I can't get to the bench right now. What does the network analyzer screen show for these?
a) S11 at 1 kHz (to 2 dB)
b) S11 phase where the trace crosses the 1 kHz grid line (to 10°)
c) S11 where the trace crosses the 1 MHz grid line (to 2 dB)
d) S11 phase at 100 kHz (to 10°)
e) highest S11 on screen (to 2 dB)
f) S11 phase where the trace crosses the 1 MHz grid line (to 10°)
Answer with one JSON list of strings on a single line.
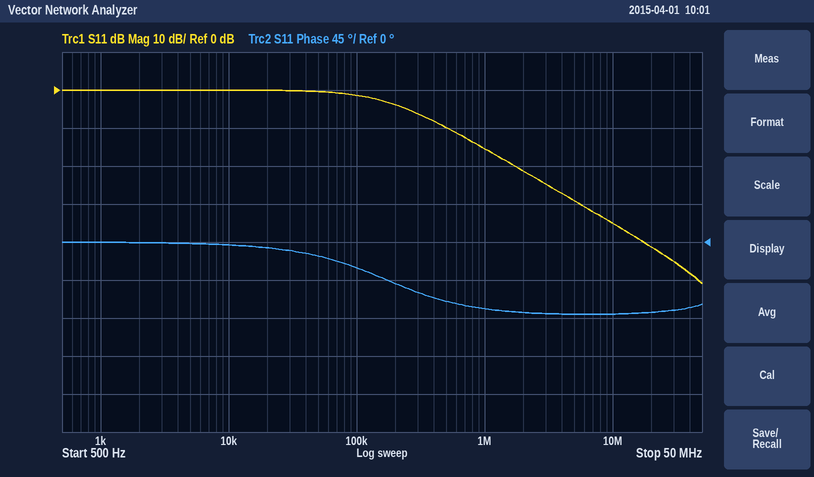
["0 dB", "0°", "-16 dB", "-30°", "0 dB", "-80°"]
